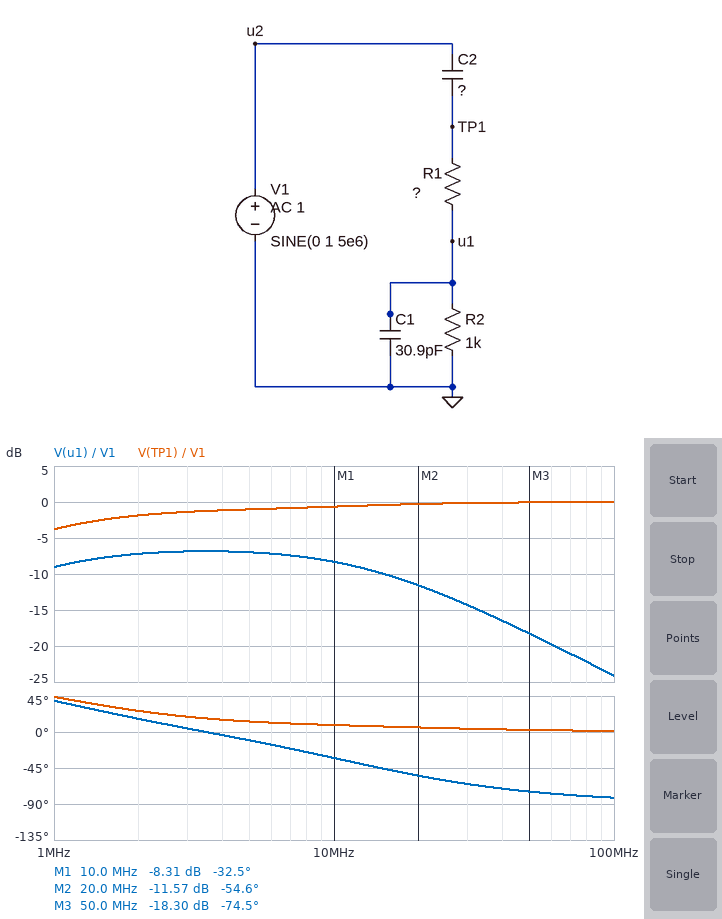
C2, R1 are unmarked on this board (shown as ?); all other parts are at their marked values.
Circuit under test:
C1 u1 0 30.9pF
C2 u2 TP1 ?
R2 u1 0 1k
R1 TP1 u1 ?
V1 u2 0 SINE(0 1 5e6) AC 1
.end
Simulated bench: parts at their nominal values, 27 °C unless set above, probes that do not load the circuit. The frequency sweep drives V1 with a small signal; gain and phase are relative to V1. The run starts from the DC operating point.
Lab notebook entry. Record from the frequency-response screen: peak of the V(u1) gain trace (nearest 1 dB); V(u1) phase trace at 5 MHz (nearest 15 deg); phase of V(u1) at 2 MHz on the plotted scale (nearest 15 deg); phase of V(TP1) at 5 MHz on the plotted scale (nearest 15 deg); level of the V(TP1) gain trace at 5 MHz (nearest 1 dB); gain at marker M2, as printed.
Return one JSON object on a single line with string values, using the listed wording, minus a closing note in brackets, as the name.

{"peak of the V(u1) gain trace": "-7 dB", "V(u1) phase trace at 5 MHz": "-15 deg", "phase of V(u1) at 2 MHz on the plotted scale": "15 deg", "phase of V(TP1) at 5 MHz on the plotted scale": "15 deg", "level of the V(TP1) gain trace at 5 MHz": "-1 dB", "gain at marker M2, as printed": "-11.57 dB"}
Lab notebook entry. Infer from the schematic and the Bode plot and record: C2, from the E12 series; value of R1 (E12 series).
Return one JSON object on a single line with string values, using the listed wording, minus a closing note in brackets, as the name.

{"C2, from the E12 series": "82 pF", "value of R1": "820 Ω"}
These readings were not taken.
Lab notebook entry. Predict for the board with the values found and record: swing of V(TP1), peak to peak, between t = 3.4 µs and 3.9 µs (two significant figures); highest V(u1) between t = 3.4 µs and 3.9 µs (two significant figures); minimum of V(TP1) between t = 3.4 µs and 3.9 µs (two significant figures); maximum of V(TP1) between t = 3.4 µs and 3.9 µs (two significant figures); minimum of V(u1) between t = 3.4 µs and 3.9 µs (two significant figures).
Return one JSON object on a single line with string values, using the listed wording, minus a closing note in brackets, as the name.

{"swing of V(TP1), peak to peak, between t = 3.4 µs and 3.9 µs": "1.8 V", "highest V(u1) between t = 3.4 µs and 3.9 µs": "450 mV", "minimum of V(TP1) between t = 3.4 µs and 3.9 µs": "-890 mV", "maximum of V(TP1) between t = 3.4 µs and 3.9 µs": "890 mV", "minimum of V(u1) between t = 3.4 µs and 3.9 µs": "-450 mV"}
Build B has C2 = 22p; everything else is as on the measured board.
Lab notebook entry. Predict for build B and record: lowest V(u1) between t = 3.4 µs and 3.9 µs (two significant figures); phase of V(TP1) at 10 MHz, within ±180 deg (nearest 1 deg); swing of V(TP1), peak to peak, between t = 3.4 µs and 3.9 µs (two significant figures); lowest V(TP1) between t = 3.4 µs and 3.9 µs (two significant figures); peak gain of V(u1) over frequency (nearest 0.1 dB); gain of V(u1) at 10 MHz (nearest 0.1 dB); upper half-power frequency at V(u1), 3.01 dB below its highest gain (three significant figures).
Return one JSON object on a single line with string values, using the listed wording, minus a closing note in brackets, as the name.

{"lowest V(u1) between t = 3.4 µs and 3.9 µs": "-300 mV", "phase of V(TP1) at 10 MHz, within ±180 deg": "26 deg", "swing of V(TP1), peak to peak, between t = 3.4 µs and 3.9 µs": "1.2 V", "lowest V(TP1) between t = 3.4 µs and 3.9 µs": "-600 mV", "peak gain of V(u1) over frequency": "-10.2 dB", "gain of V(u1) at 10 MHz": "-10.5 dB", "upper half-power frequency at V(u1), 3.01 dB below its highest gain": "22.3 MHz"}
